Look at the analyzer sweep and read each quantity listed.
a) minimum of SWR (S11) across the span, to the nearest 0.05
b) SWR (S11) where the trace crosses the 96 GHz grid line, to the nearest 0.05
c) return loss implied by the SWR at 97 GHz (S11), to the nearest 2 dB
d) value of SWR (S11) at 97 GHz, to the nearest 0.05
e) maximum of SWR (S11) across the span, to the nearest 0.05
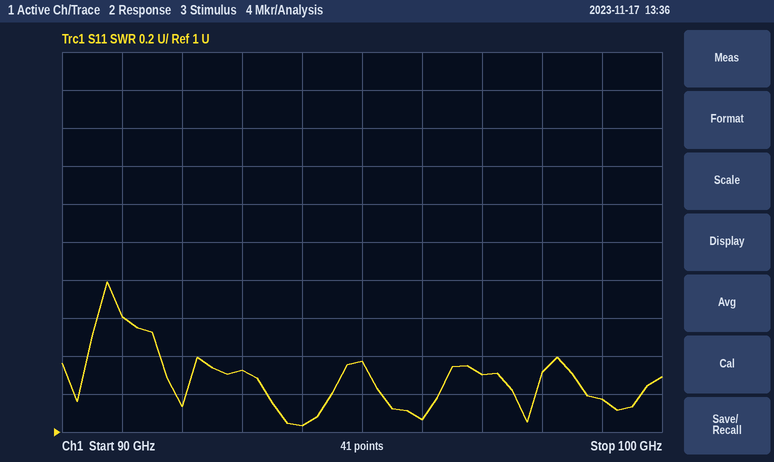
1.05
1.05
18 dB
1.30
1.80
